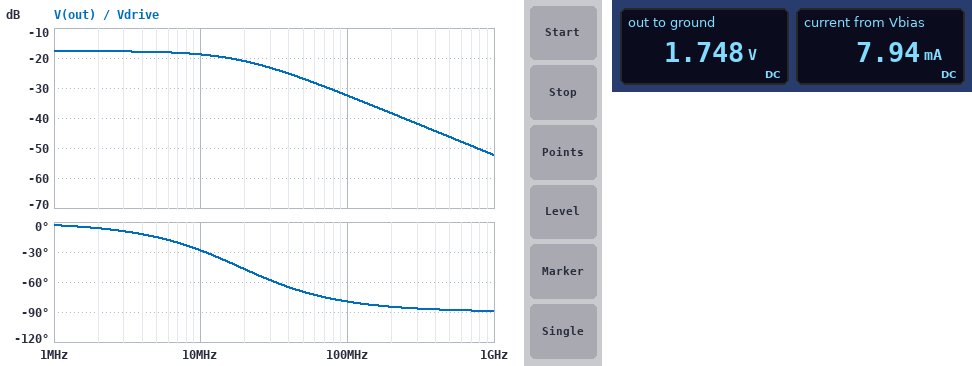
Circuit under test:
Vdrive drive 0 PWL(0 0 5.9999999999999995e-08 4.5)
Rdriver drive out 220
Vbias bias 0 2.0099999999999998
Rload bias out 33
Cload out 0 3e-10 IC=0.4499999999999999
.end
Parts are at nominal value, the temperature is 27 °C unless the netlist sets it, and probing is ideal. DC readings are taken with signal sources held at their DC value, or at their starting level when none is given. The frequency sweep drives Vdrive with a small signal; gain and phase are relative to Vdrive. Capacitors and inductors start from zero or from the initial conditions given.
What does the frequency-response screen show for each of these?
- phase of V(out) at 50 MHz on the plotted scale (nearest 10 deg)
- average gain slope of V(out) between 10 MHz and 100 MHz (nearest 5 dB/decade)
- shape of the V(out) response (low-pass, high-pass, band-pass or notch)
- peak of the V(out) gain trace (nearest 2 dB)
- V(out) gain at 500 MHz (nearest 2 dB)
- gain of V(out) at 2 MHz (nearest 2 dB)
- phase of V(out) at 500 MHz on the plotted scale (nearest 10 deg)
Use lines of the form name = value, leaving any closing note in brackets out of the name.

phase of V(out) at 50 MHz on the plotted scale = -70 deg
average gain slope of V(out) between 10 MHz and 100 MHz = -15 dB/decade
shape of the V(out) response = low-pass
peak of the V(out) gain trace = -18 dB
V(out) gain at 500 MHz = -46 dB
gain of V(out) at 2 MHz = -18 dB
phase of V(out) at 500 MHz on the plotted scale = -90 deg
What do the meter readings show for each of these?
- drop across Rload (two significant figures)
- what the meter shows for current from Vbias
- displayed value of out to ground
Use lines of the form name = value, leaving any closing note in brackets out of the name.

drop across Rload = 260 mV
what the meter shows for current from Vbias = 7.94 mA
displayed value of out to ground = 1.748 V
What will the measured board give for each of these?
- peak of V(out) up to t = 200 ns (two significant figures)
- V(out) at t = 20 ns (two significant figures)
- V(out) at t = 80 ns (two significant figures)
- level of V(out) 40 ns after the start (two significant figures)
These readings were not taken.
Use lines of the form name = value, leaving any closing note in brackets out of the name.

peak of V(out) up to t = 200 ns = 2.3 V
V(out) at t = 20 ns = 1.7 V
V(out) at t = 80 ns = 2.3 V
level of V(out) 40 ns after the start = 2.0 V
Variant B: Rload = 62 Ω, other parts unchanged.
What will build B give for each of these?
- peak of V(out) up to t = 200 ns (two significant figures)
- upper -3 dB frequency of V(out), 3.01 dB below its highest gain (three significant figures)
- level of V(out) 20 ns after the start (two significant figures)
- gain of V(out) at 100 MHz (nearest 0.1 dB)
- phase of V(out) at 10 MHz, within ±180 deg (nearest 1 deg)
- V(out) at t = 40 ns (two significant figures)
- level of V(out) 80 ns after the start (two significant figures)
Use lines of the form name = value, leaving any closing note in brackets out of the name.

peak of V(out) up to t = 200 ns = 2.6 V
upper -3 dB frequency of V(out), 3.01 dB below its highest gain = 11.0 MHz
level of V(out) 20 ns after the start = 1.4 V
gain of V(out) at 100 MHz = -32.4 dB
phase of V(out) at 10 MHz, within ±180 deg = -42 deg
V(out) at t = 40 ns = 1.9 V
level of V(out) 80 ns after the start = 2.5 V
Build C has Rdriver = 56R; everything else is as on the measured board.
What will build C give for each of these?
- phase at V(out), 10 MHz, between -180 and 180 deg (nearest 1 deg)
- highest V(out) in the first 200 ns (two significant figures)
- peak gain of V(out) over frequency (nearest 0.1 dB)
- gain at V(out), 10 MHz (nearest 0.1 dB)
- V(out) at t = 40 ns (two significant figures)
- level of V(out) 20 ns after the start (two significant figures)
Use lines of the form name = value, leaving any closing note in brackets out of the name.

phase at V(out), 10 MHz, between -180 and 180 deg = -21 deg
highest V(out) in the first 200 ns = 2.9 V
peak gain of V(out) over frequency = -8.6 dB
gain at V(out), 10 MHz = -9.2 dB
V(out) at t = 40 ns = 2.2 V
level of V(out) 20 ns after the start = 1.6 V
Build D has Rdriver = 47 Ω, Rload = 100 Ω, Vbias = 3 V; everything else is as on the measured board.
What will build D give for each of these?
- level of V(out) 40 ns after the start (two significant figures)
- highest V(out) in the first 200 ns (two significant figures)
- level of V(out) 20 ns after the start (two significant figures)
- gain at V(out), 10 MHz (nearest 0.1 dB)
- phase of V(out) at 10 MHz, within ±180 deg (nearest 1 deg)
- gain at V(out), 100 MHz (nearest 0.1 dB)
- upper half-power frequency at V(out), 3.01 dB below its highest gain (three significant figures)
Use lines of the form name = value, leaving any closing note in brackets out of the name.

level of V(out) 40 ns after the start = 2.5 V
highest V(out) in the first 200 ns = 4.0 V
level of V(out) 20 ns after the start = 1.5 V
gain at V(out), 10 MHz = -4.7 dB
phase of V(out) at 10 MHz, within ±180 deg = -31 deg
gain at V(out), 100 MHz = -19.1 dB
upper half-power frequency at V(out), 3.01 dB below its highest gain = 16.6 MHz
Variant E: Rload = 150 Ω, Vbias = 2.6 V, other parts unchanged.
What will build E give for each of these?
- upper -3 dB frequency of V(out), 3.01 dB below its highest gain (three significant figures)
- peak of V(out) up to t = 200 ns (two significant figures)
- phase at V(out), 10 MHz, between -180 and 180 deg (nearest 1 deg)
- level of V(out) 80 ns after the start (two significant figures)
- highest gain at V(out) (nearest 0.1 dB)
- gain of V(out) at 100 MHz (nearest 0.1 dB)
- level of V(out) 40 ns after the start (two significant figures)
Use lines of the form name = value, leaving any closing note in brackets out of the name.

upper -3 dB frequency of V(out), 3.01 dB below its highest gain = 5.95 MHz
peak of V(out) up to t = 200 ns = 3.4 V
phase at V(out), 10 MHz, between -180 and 180 deg = -59 deg
level of V(out) 80 ns after the start = 3.0 V
highest gain at V(out) = -7.8 dB
gain of V(out) at 100 MHz = -32.4 dB
level of V(out) 40 ns after the start = 1.9 V
